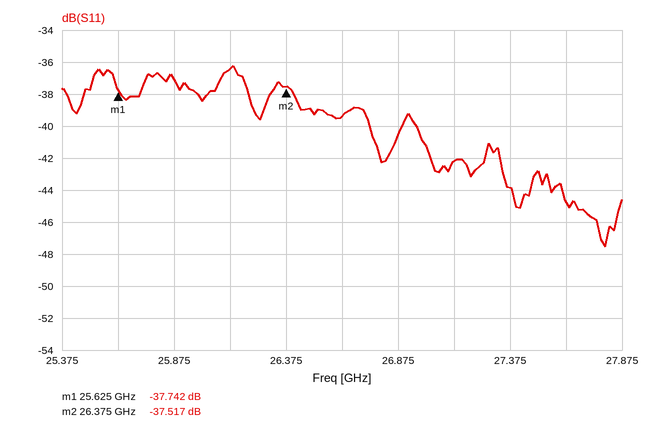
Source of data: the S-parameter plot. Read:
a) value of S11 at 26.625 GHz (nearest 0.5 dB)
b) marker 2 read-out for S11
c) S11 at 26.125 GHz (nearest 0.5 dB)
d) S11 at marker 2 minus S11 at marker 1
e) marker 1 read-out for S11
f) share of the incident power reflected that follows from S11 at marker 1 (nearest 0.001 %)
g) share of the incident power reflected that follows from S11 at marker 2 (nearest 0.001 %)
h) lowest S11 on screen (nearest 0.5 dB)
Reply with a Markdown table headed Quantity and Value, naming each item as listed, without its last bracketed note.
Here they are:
| Quantity | Value |
|---|---|
| value of S11 at 26.625 GHz | -39.5 dB |
| marker 2 read-out for S11 | -37.517 dB |
| S11 at 26.125 GHz | -36.5 dB |
| S11 at marker 2 minus S11 at marker 1 | 0.225 dB |
| marker 1 read-out for S11 | -37.742 dB |
| share of the incident power reflected that follows from S11 at marker 1 | 0.017 % |
| share of the incident power reflected that follows from S11 at marker 2 | 0.018 % |
| lowest S11 on screen | -47.5 dB |
